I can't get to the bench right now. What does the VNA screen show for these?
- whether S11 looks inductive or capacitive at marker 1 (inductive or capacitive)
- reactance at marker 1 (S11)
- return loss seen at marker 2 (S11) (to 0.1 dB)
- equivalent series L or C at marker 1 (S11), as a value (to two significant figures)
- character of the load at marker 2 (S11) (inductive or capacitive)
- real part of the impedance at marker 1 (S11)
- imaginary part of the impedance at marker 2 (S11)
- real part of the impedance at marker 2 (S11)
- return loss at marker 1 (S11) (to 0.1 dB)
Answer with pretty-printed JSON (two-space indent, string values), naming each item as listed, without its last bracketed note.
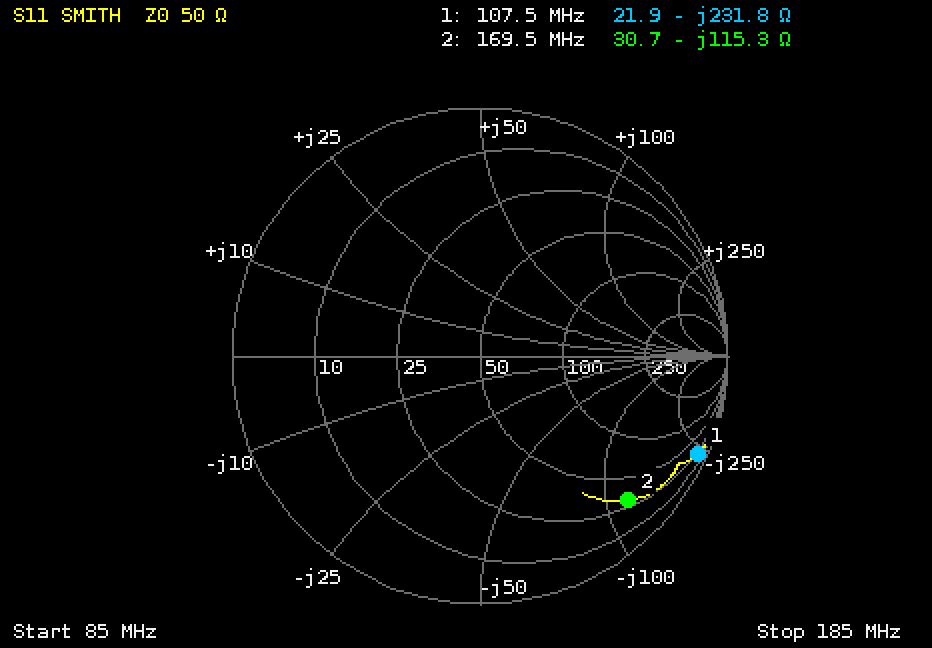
{
  "whether S11 looks inductive or capacitive at marker 1": "capacitive",
  "reactance at marker 1": "-231.8 Ω",
  "return loss seen at marker 2 (S11)": "1.6 dB",
  "equivalent series L or C at marker 1 (S11), as a value": "6.4 pF",
  "character of the load at marker 2 (S11)": "capacitive",
  "real part of the impedance at marker 1": "21.9 Ω",
  "imaginary part of the impedance at marker 2": "-115.3 Ω",
  "real part of the impedance at marker 2": "30.7 Ω",
  "return loss at marker 1 (S11)": "0.3 dB"
}
